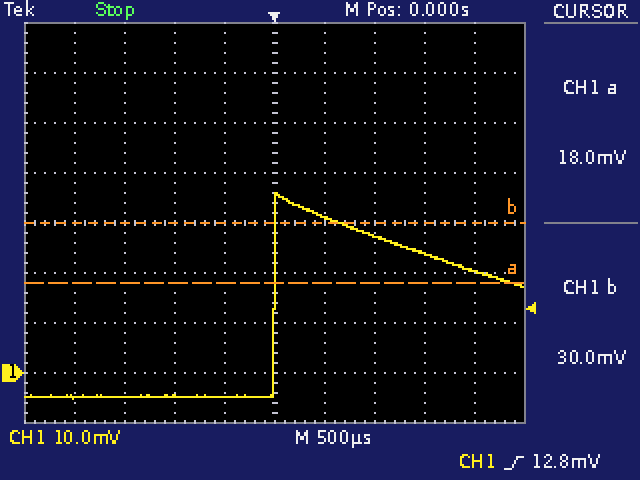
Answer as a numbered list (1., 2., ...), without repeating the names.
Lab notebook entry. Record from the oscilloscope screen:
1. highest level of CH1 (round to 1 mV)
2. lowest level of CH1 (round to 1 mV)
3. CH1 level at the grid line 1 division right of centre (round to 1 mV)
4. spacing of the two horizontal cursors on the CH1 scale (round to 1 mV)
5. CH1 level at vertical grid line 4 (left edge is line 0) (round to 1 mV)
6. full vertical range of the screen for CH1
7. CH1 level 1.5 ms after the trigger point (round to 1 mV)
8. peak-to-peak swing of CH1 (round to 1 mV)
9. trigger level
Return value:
1. 36 mV
2. -5 mV
3. 31 mV
4. 12 mV
5. -5 mV
6. 80 mV
7. 24 mV
8. 41 mV
9. 12.8 mV
